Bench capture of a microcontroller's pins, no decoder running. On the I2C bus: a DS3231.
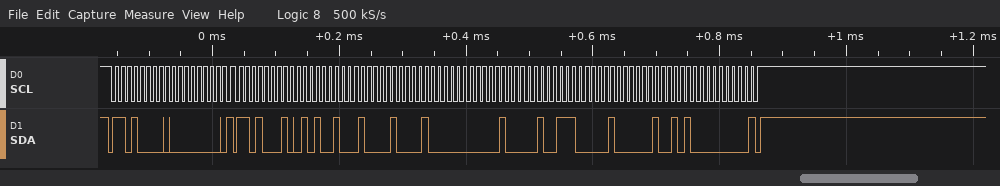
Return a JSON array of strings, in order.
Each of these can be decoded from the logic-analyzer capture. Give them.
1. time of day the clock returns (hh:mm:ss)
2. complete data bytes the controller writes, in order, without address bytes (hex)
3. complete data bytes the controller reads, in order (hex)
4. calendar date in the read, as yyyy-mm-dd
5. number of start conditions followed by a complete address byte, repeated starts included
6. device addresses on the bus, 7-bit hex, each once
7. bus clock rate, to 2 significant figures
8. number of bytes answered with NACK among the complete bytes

["20:42:52", "00", "52 42 20 04 27 08 25 00", "2025-08-27", "2", "0x68", "100 kHz", "1"]
